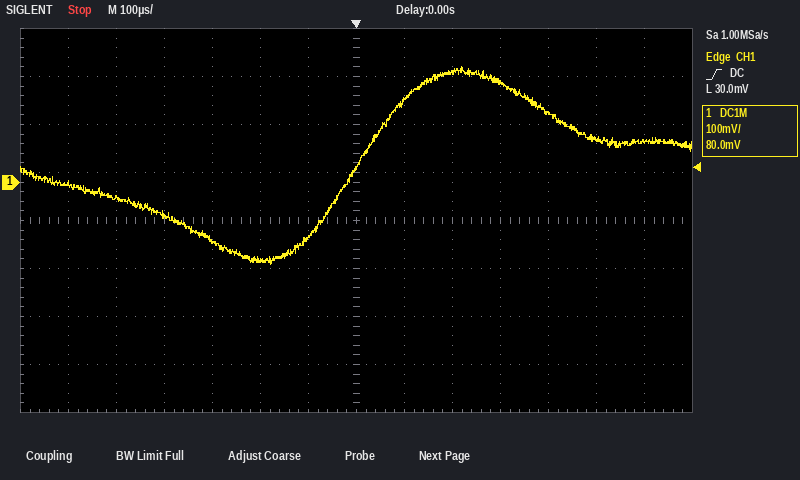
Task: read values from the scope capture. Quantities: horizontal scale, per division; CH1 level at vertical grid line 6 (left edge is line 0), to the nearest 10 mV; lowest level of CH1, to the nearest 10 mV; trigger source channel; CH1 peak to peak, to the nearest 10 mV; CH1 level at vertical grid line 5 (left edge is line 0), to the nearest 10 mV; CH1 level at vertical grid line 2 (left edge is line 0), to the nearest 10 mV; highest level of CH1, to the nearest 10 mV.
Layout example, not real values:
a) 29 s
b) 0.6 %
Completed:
a) 100 µs
b) -120 mV
c) -170 mV
d) CH1
e) 410 mV
f) -160 mV
g) -30 mV
h) 240 mV
